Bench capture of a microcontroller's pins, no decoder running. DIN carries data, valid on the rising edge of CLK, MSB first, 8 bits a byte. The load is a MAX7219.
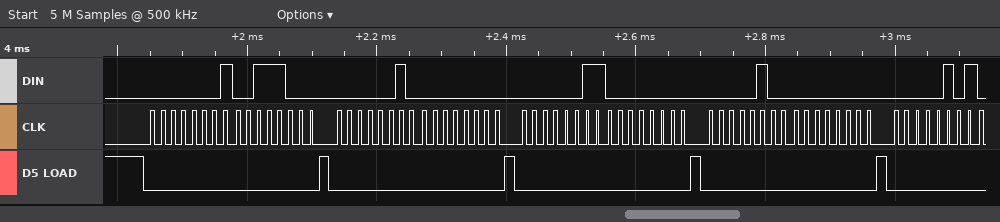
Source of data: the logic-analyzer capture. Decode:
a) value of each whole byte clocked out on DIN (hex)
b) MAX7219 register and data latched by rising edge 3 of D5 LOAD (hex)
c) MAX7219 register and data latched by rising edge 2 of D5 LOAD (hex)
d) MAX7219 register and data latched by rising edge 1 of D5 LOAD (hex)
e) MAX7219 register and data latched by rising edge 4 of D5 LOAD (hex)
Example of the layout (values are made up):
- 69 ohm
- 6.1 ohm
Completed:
- 0x01 0x38 0x02 0x00 0x03 0x00 0x04 0x00 0x05
- register 0x3, data 0x00
- register 0x2, data 0x00
- register 0x1, data 0x38
- register 0x4, data 0x00
